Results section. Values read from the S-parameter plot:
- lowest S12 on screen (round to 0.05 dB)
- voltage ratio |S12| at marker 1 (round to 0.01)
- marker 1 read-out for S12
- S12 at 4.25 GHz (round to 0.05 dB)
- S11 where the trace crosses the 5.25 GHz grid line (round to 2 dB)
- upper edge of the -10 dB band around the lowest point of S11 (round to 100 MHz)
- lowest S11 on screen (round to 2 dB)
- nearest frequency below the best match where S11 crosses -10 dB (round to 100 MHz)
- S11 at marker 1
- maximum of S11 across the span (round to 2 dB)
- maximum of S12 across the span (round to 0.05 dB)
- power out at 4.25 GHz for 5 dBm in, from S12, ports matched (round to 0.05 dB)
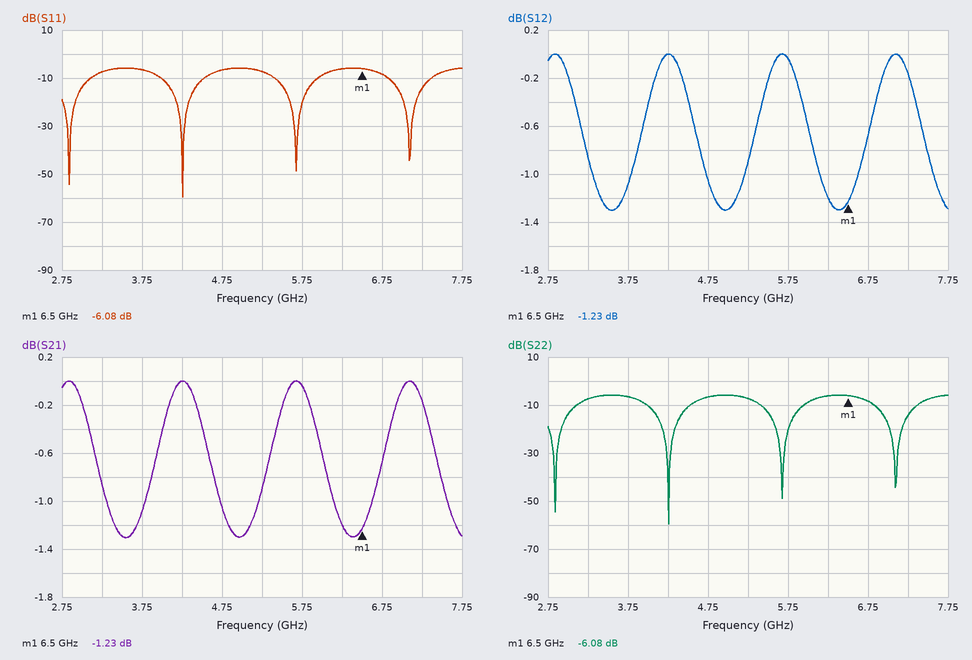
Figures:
-1.30 dB
0.87
-1.23 dB
0.00 dB
-8 dB
4.5 GHz
-60 dB
4.0 GHz
-6.08 dB
-6 dB
0.00 dB
5.00 dBm
